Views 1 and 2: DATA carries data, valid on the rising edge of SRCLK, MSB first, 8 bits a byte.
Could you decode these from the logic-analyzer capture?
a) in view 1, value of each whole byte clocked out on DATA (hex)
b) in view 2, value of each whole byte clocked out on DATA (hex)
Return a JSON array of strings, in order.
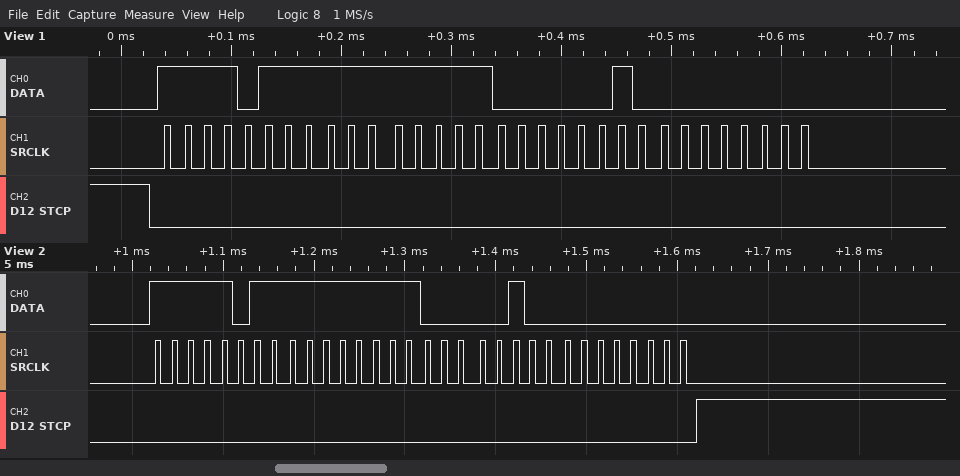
["F7 FF 02 00", "FB FF 04 00"]
